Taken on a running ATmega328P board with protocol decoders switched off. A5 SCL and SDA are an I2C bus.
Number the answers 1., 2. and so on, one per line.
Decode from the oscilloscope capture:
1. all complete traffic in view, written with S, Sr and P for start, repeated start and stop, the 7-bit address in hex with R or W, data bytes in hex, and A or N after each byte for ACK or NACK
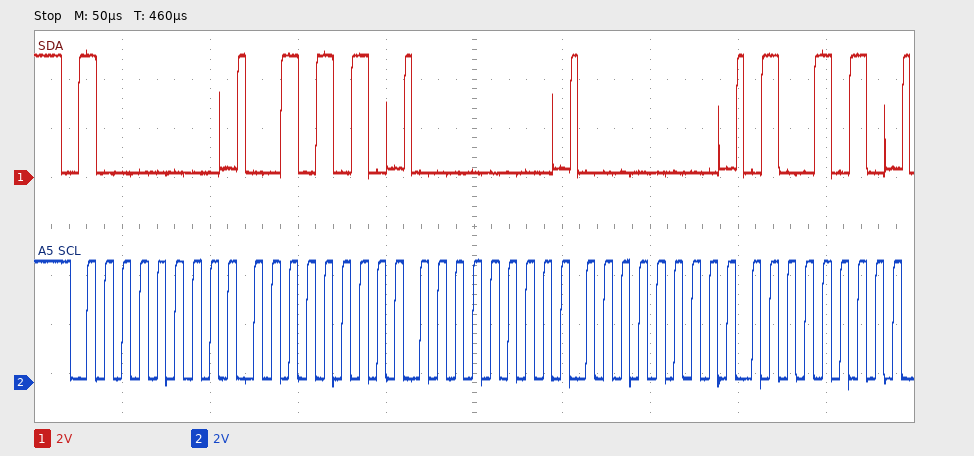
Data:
1. S 40W A 2A A 00 A 00 A 4A A
